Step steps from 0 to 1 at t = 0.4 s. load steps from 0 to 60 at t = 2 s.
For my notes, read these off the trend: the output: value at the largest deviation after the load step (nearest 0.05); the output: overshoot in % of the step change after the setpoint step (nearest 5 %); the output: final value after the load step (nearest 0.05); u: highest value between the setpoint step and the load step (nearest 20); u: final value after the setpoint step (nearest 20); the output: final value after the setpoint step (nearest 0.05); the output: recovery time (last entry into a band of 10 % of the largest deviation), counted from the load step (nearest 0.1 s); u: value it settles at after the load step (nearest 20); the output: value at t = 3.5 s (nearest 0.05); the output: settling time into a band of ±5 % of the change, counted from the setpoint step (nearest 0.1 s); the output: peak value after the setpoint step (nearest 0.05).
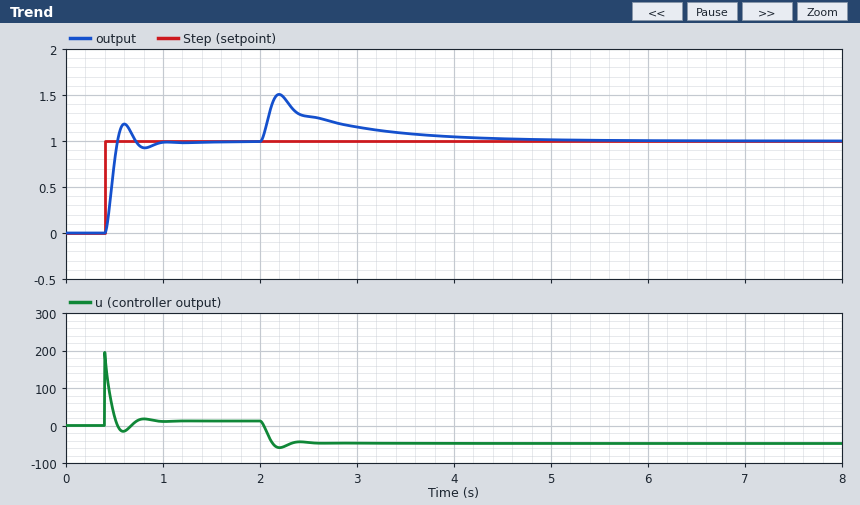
1.50
20 %
1.00
200
20
1.00
1.9 s
-40
1.10
0.5 s
1.20
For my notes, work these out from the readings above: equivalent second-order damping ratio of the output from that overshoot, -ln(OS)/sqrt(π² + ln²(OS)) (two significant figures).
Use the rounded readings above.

0.46
